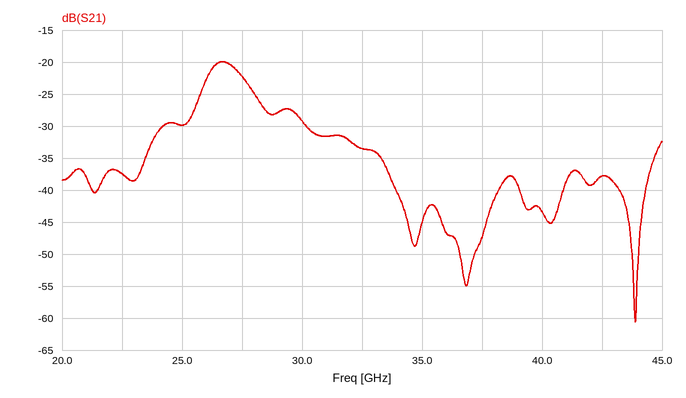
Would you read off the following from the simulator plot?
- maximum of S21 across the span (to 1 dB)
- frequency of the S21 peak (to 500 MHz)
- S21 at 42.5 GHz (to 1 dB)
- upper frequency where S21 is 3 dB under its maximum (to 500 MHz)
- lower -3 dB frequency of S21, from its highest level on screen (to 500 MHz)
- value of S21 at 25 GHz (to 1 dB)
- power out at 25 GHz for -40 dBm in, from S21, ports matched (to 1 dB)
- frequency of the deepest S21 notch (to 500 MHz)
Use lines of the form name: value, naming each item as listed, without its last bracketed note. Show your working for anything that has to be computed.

maximum of S21 across the span: -20 dB
frequency of the S21 peak: 26.5 GHz
S21 at 42.5 GHz: -38 dB
upper frequency where S21 is 3 dB under its maximum: 27.5 GHz
lower -3 dB frequency of S21, from its highest level on screen: 26.0 GHz
value of S21 at 25 GHz: -30 dB
power out at 25 GHz for -40 dBm in, from S21, ports matched: -40 dBm + (-30 dB) = -70 dBm
frequency of the deepest S21 notch: 44.0 GHz
